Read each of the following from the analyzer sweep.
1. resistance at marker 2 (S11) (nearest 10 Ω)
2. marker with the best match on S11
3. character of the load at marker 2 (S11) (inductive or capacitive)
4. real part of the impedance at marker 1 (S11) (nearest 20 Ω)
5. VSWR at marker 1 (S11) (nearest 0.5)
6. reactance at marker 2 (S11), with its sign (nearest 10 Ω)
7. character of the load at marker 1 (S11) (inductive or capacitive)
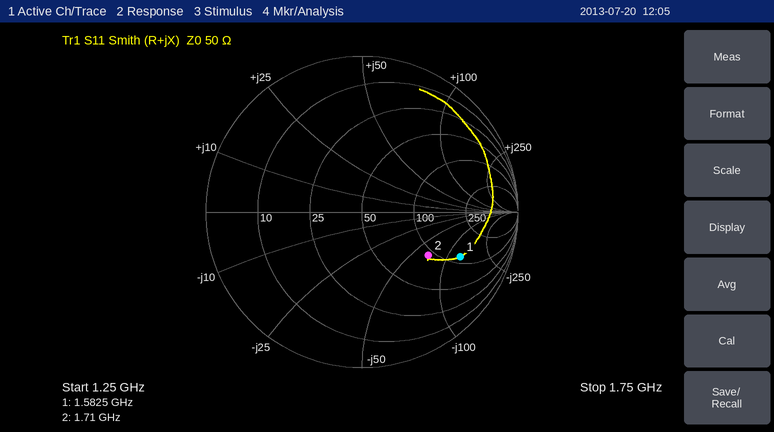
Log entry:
90 Ω
marker 2
capacitive
120 Ω
5.5
-70 Ω
capacitive
